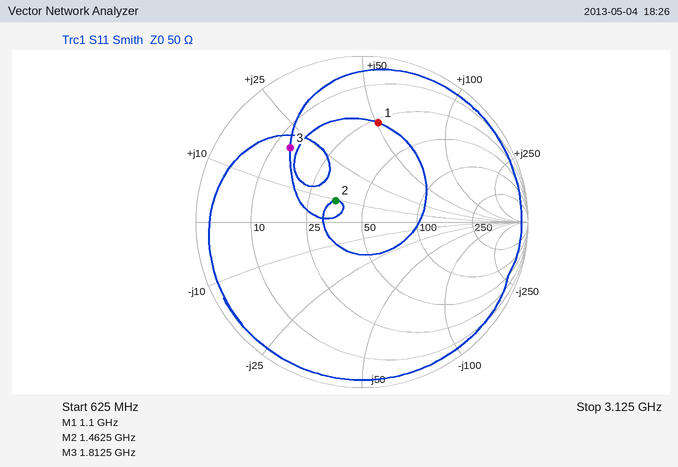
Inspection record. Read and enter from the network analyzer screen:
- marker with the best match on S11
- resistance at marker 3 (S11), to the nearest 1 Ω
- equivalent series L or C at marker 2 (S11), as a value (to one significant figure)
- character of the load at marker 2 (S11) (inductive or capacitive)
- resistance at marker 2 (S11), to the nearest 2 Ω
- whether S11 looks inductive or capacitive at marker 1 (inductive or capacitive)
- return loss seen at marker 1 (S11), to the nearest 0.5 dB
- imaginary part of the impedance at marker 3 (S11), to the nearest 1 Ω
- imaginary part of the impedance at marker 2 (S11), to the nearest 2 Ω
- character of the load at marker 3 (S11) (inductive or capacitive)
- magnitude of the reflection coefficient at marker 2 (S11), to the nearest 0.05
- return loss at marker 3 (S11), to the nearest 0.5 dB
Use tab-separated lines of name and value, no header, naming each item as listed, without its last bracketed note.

marker with the best match on S11	marker 2
resistance at marker 3 (S11), to the nearest 1 Ω	14 Ω
equivalent series L or C at marker 2 (S11), as a value	1 nH
character of the load at marker 2 (S11)	inductive
resistance at marker 2 (S11), to the nearest 2 Ω	36 Ω
whether S11 looks inductive or capacitive at marker 1	inductive
return loss seen at marker 1 (S11), to the nearest 0.5 dB	4.5 dB
imaginary part of the impedance at marker 3 (S11), to the nearest 1 Ω	+20 Ω
imaginary part of the impedance at marker 2 (S11), to the nearest 2 Ω	+10 Ω
character of the load at marker 3 (S11)	inductive
magnitude of the reflection coefficient at marker 2 (S11), to the nearest 0.05	0.20
return loss at marker 3 (S11), to the nearest 0.5 dB	4.0 dB
